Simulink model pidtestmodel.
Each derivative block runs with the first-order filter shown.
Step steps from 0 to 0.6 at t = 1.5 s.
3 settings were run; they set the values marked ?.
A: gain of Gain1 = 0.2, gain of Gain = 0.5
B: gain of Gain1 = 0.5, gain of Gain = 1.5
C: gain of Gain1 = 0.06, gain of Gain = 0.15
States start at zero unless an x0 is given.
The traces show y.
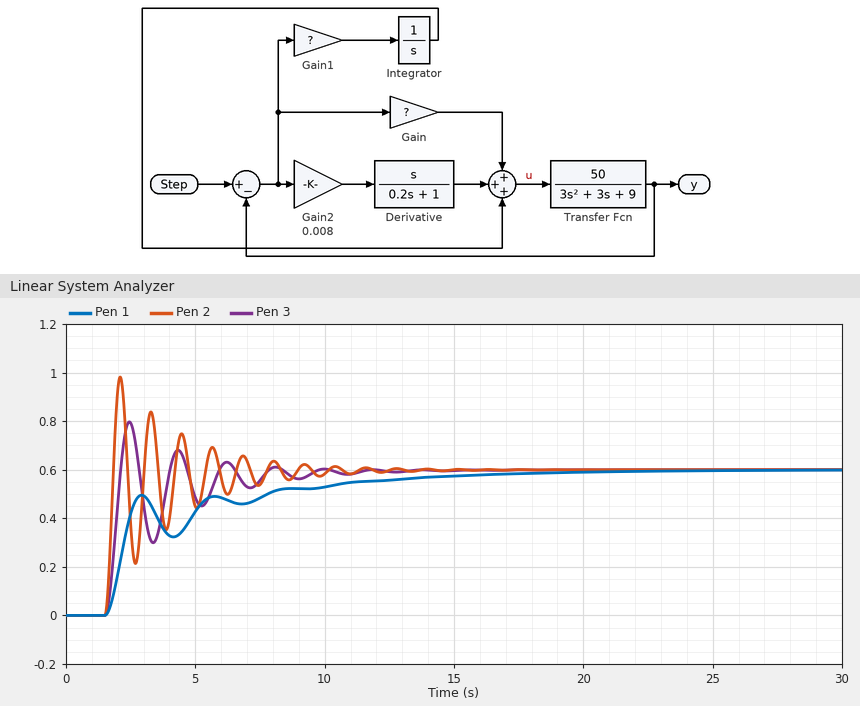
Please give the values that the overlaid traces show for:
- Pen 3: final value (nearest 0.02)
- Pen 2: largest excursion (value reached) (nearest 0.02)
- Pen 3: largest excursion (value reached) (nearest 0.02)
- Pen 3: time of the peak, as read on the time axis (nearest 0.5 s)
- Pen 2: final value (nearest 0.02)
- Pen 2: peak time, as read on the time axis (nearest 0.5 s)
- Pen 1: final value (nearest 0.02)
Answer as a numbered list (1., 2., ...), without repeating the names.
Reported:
1. 0.60
2. 0.98
3. 0.80
4. 2.5 s
5. 0.60
6. 2.0 s
7. 0.60
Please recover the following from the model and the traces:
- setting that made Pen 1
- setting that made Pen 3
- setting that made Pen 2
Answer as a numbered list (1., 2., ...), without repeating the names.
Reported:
1. C
2. A
3. B
